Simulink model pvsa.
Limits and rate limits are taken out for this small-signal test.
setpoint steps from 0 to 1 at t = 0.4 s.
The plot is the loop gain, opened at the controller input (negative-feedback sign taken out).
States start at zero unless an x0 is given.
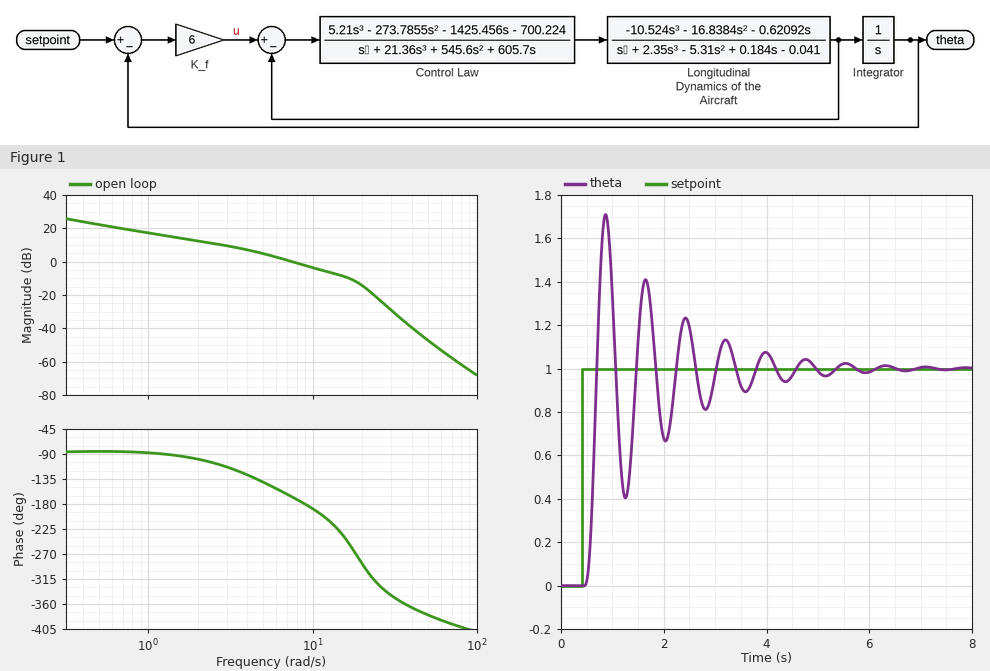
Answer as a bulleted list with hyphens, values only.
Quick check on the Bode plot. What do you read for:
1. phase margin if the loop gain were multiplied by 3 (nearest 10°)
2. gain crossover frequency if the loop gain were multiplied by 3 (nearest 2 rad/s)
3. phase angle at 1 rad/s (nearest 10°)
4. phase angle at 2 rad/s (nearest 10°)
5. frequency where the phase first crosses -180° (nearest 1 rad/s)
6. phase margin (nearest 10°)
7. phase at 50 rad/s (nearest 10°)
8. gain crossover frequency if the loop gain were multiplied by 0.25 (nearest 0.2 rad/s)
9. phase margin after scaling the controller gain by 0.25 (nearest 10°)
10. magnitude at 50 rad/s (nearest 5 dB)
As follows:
- -70°
- 16 rad/s
- -90°
- -100°
- 9 rad/s
- 10°
- -380°
- 2.2 rad/s
- 80°
- -45 dB
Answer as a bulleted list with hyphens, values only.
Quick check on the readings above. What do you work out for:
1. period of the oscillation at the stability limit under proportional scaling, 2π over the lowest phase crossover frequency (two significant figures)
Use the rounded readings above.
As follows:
- 0.70 s
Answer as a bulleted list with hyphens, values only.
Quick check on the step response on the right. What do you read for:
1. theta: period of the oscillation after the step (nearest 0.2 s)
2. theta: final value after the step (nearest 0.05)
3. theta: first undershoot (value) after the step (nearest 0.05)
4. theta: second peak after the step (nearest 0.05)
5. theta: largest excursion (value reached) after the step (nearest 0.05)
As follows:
- 0.8 s
- 1.00
- 0.40
- 1.40
- 1.70
